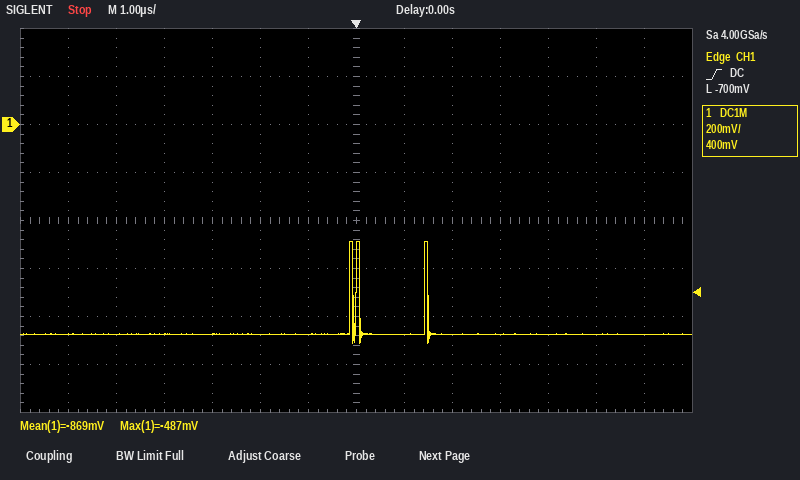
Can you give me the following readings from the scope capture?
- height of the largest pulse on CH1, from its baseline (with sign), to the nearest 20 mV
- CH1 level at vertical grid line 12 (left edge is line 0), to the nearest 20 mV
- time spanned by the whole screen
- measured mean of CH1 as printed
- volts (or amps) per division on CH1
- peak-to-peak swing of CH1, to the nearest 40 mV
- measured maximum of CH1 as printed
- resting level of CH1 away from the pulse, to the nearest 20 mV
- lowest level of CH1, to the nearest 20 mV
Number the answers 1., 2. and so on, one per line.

1. +380 mV
2. -880 mV
3. 14 µs
4. -869 mV
5. 200 mV
6. 440 mV
7. -487 mV
8. -880 mV
9. -920 mV
